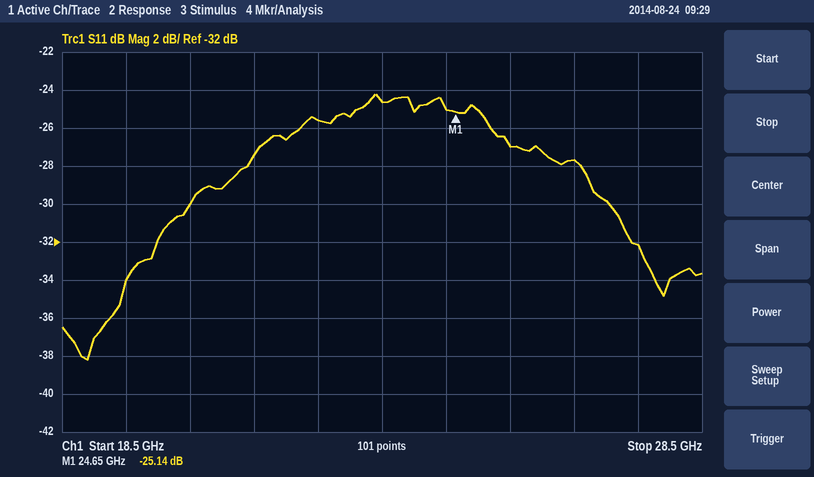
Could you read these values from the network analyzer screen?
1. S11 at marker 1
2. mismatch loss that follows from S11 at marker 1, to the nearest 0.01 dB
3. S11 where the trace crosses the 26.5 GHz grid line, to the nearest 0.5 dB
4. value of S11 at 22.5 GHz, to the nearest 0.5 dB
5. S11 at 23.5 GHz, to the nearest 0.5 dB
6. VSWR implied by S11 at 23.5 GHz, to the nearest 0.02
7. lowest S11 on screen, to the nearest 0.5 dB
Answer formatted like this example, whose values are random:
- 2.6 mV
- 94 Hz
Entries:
- -25.14 dB
- 0.01 dB
- -27.5 dB
- -25.5 dB
- -24.5 dB
- 1.12
- -38.0 dB
